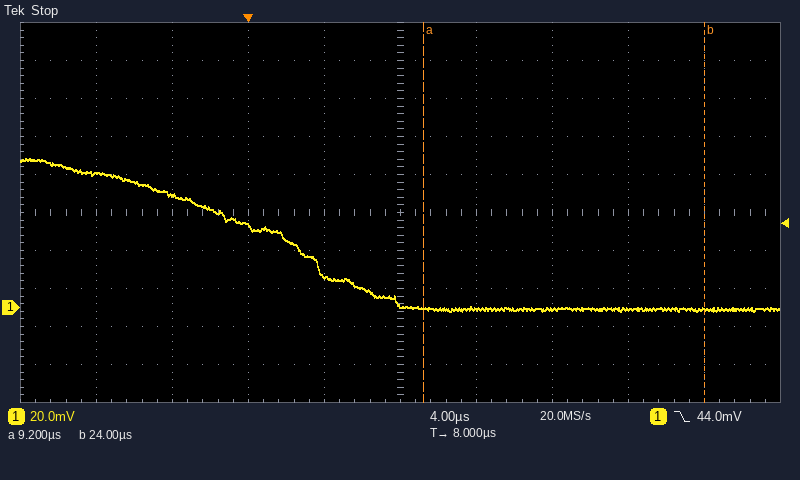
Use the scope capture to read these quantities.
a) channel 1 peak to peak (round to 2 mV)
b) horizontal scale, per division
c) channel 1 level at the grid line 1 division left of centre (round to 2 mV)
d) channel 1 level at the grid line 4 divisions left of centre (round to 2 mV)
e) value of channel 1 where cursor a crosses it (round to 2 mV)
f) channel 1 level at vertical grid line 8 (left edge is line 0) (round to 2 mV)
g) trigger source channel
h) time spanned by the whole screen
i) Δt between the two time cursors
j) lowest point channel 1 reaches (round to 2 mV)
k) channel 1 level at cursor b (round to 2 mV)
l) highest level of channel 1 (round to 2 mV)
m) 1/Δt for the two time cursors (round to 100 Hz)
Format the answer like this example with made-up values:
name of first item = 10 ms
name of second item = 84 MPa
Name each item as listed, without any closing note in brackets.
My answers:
channel 1 peak to peak = 80 mV
horizontal scale, per division = 4 µs
channel 1 level at the grid line 1 division left of centre = 16 mV
channel 1 level at the grid line 4 divisions left of centre = 70 mV
value of channel 1 where cursor a crosses it = 0 mV
channel 1 level at vertical grid line 8 (left edge is line 0) = 0 mV
trigger source channel = channel 1
time spanned by the whole screen = 40 µs
Δt between the two time cursors = 14.8 µs
lowest point channel 1 reaches = -2 mV
channel 1 level at cursor b = 0 mV
highest level of channel 1 = 78 mV
1/Δt for the two time cursors = 67.6 kHz
